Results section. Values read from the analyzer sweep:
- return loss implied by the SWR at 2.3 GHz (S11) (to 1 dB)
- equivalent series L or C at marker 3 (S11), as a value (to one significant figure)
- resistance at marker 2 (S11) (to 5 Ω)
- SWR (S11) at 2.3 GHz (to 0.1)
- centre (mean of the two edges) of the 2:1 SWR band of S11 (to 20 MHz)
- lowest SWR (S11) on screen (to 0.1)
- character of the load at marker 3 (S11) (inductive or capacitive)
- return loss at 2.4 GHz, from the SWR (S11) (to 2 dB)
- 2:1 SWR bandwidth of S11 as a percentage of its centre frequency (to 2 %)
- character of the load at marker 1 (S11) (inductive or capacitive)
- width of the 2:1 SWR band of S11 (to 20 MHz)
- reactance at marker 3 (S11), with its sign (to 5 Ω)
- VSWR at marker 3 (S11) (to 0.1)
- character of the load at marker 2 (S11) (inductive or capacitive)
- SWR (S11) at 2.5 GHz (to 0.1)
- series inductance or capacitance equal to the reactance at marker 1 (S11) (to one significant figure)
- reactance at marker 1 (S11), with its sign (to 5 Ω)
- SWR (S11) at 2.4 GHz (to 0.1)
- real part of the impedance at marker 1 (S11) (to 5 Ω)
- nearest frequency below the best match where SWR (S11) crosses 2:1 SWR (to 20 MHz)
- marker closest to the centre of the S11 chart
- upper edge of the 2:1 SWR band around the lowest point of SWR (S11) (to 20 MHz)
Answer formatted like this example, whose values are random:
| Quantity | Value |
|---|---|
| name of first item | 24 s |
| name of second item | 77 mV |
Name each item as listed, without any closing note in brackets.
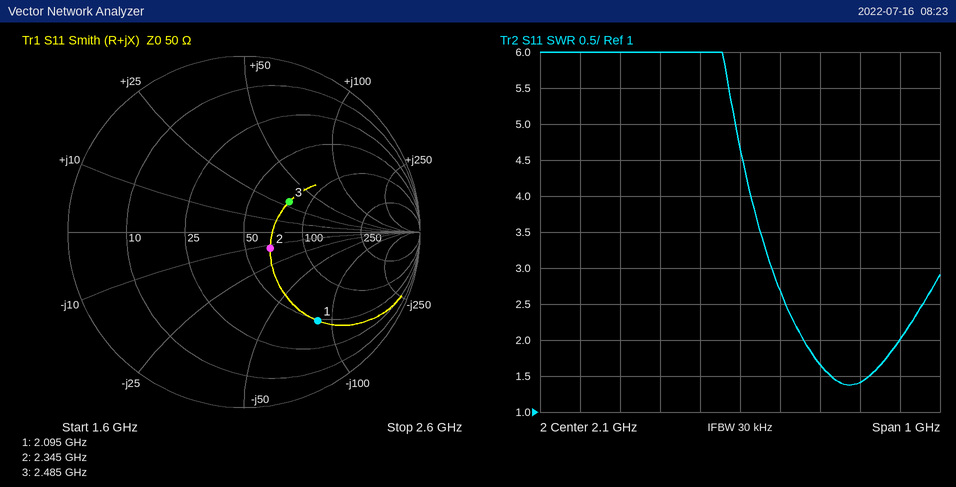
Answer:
| Quantity | Value |
|---|---|
| return loss implied by the SWR at 2.3 GHz (S11) | 12 dB |
| equivalent series L or C at marker 3 (S11), as a value | 2 nH |
| resistance at marker 2 (S11) | 65 Ω |
| SWR (S11) at 2.3 GHz | 1.7 |
| centre (mean of the two edges) of the 2:1 SWR band of S11 | 2.38 GHz |
| lowest SWR (S11) on screen | 1.4 |
| character of the load at marker 3 (S11) | inductive |
| return loss at 2.4 GHz, from the SWR (S11) | 16 dB |
| 2:1 SWR bandwidth of S11 as a percentage of its centre frequency | 10 % |
| character of the load at marker 1 (S11) | capacitive |
| width of the 2:1 SWR band of S11 | 240 MHz |
| reactance at marker 3 (S11), with its sign | +30 Ω |
| VSWR at marker 3 (S11) | 1.9 |
| character of the load at marker 2 (S11) | capacitive |
| SWR (S11) at 2.5 GHz | 2.0 |
| series inductance or capacitance equal to the reactance at marker 1 (S11) | 900 fF |
| reactance at marker 1 (S11), with its sign | -85 Ω |
| SWR (S11) at 2.4 GHz | 1.4 |
| real part of the impedance at marker 1 (S11) | 50 Ω |
| nearest frequency below the best match where SWR (S11) crosses 2:1 SWR | 2.26 GHz |
| marker closest to the centre of the S11 chart | marker 2 |
| upper edge of the 2:1 SWR band around the lowest point of SWR (S11) | 2.50 GHz |
